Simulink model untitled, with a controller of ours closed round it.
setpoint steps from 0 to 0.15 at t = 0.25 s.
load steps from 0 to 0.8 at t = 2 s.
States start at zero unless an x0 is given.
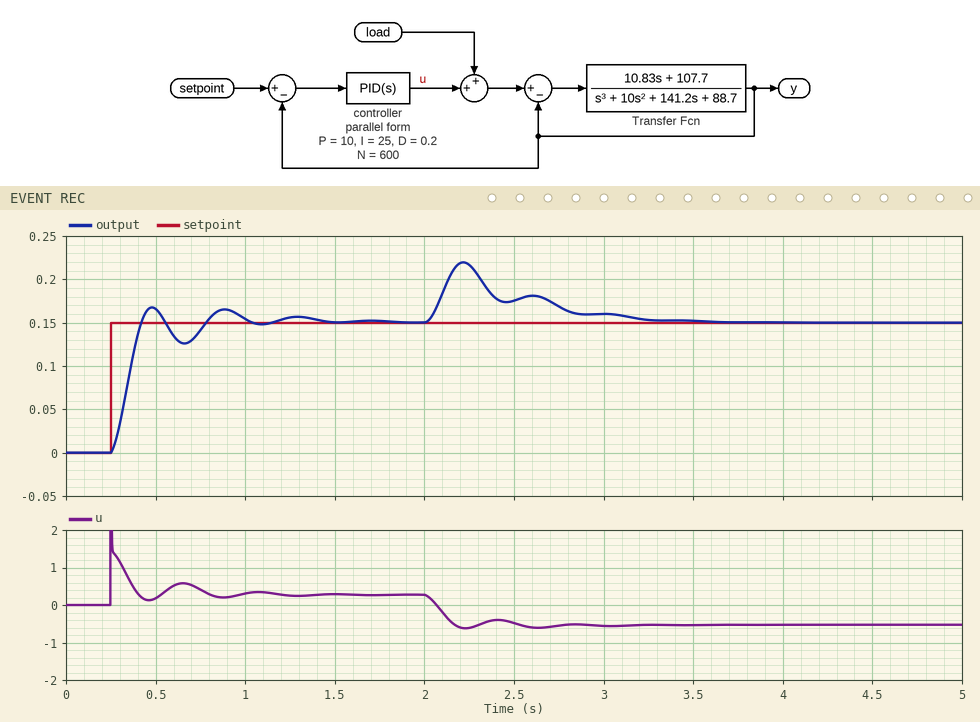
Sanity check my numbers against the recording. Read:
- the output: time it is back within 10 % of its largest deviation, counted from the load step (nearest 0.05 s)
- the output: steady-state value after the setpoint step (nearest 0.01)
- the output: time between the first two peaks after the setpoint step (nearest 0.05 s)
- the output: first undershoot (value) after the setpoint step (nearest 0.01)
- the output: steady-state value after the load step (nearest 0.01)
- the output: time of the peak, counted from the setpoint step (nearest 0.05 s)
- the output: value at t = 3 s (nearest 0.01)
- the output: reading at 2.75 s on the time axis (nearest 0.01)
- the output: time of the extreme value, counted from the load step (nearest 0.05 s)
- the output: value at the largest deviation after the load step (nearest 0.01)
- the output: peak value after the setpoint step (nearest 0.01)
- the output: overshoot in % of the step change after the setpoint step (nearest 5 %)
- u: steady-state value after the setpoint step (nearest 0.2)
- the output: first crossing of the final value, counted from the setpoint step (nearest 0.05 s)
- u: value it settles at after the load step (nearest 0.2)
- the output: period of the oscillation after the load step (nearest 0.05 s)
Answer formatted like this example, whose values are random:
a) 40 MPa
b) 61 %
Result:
a) 1.15 s
b) 0.15
c) 0.40 s
d) 0.13
e) 0.15
f) 0.25 s
g) 0.16
h) 0.17
i) 0.20 s
j) 0.22
k) 0.17
l) 10 %
m) 0.2
n) 0.15 s
o) -0.6
p) 0.40 s
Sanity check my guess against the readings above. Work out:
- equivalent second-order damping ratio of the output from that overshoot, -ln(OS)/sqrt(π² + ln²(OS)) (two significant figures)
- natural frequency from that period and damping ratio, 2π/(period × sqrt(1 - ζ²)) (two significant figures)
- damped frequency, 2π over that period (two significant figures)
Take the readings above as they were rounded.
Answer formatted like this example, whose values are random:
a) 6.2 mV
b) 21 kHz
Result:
a) 0.59
b) 19 rad/s
c) 16 rad/s
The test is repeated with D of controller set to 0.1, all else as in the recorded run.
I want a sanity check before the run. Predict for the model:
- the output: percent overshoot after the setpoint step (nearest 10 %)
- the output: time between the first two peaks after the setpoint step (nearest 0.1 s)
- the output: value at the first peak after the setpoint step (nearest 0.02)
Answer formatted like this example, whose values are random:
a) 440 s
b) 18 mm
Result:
a) 20 %
b) 0.4 s
c) 0.18
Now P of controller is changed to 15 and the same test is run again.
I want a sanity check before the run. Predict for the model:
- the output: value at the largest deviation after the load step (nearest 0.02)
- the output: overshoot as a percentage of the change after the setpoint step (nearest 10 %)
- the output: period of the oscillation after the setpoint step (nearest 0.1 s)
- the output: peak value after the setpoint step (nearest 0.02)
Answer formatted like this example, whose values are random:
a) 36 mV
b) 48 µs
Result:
a) 0.20
b) 20 %
c) 0.4 s
d) 0.18
